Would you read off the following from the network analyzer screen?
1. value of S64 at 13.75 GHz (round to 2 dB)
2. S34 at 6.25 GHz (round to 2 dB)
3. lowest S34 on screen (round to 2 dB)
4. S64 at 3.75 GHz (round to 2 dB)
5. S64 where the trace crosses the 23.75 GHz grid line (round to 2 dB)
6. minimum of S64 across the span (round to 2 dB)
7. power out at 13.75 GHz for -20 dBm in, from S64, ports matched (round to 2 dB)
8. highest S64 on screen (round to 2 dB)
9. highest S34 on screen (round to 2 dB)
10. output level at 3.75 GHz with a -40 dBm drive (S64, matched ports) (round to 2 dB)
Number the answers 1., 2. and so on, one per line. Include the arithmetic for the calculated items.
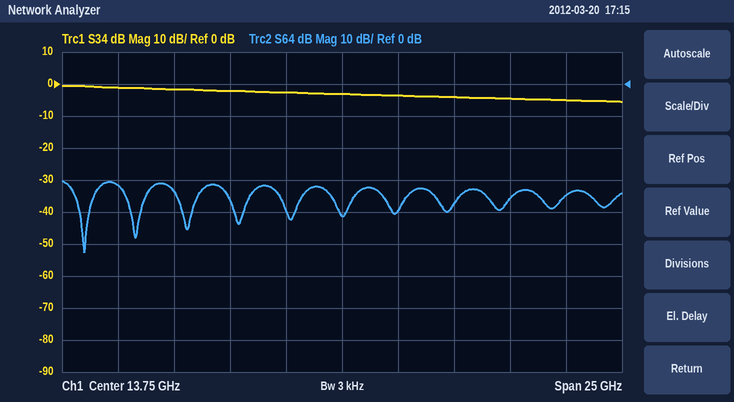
1. -42 dB
2. -2 dB
3. -6 dB
4. -32 dB
5. -34 dB
6. -52 dB
7. -20 dBm + (-42 dB) = -62 dBm
8. -30 dB
9. 0 dB
10. -40 dBm + (-32 dB) = -72 dBm
